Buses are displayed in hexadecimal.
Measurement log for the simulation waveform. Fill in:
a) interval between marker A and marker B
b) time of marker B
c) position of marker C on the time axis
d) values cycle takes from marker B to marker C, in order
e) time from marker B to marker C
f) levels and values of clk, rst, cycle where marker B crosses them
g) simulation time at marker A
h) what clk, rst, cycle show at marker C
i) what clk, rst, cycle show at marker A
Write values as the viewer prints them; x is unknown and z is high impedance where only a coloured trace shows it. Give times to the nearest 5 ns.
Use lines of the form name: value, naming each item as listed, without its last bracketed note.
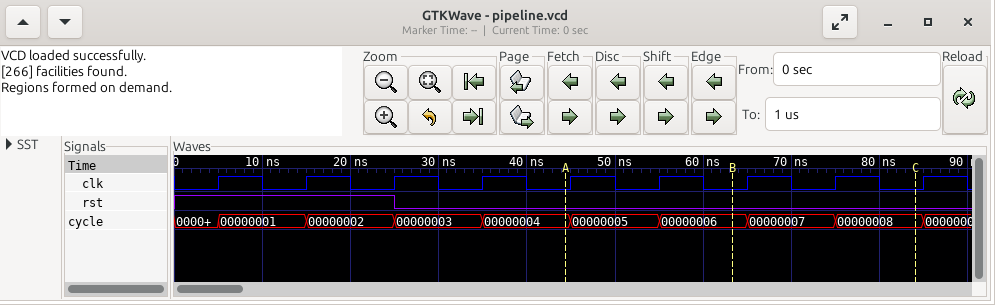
interval between marker A and marker B: 20 ns
time of marker B: 65 ns
position of marker C on the time axis: 85 ns
values cycle takes from marker B to marker C, in order: 00000006, 00000007, 00000008
time from marker B to marker C: 20 ns
levels and values of clk, rst, cycle where marker B crosses them: clk=0, rst=0, cycle=00000006
simulation time at marker A: 45 ns
what clk, rst, cycle show at marker C: clk=0, rst=0, cycle=00000008
what clk, rst, cycle show at marker A: clk=0, rst=0, cycle=00000004
